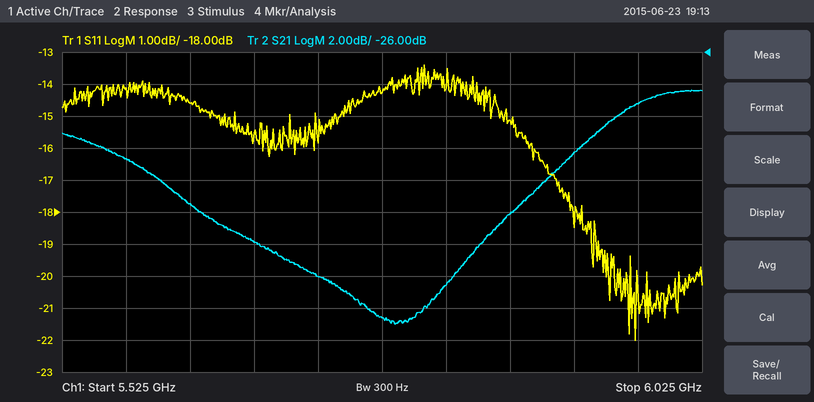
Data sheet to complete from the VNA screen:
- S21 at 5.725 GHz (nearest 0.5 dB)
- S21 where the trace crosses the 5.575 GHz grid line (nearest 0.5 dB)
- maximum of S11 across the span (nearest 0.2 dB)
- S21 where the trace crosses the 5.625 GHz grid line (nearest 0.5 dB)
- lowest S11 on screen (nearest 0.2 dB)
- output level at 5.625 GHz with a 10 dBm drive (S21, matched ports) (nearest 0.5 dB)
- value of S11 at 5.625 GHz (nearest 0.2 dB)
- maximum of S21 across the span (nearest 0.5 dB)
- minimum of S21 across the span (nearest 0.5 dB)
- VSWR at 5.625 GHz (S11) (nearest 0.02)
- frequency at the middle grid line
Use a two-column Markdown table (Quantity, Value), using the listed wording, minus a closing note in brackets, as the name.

| Quantity | Value |
|---|---|
| S21 at 5.725 GHz | -40.0 dB |
| S21 where the trace crosses the 5.575 GHz grid line | -32.5 dB |
| maximum of S11 across the span | -13.4 dB |
| S21 where the trace crosses the 5.625 GHz grid line | -35.5 dB |
| lowest S11 on screen | -22.0 dB |
| output level at 5.625 GHz with a 10 dBm drive (S21, matched ports) | -25.5 dBm |
| value of S11 at 5.625 GHz | -14.6 dB |
| maximum of S21 across the span | -28.5 dB |
| minimum of S21 across the span | -43.0 dB |
| VSWR at 5.625 GHz (S11) | 1.46 |
| frequency at the middle grid line | 5.775 GHz |
